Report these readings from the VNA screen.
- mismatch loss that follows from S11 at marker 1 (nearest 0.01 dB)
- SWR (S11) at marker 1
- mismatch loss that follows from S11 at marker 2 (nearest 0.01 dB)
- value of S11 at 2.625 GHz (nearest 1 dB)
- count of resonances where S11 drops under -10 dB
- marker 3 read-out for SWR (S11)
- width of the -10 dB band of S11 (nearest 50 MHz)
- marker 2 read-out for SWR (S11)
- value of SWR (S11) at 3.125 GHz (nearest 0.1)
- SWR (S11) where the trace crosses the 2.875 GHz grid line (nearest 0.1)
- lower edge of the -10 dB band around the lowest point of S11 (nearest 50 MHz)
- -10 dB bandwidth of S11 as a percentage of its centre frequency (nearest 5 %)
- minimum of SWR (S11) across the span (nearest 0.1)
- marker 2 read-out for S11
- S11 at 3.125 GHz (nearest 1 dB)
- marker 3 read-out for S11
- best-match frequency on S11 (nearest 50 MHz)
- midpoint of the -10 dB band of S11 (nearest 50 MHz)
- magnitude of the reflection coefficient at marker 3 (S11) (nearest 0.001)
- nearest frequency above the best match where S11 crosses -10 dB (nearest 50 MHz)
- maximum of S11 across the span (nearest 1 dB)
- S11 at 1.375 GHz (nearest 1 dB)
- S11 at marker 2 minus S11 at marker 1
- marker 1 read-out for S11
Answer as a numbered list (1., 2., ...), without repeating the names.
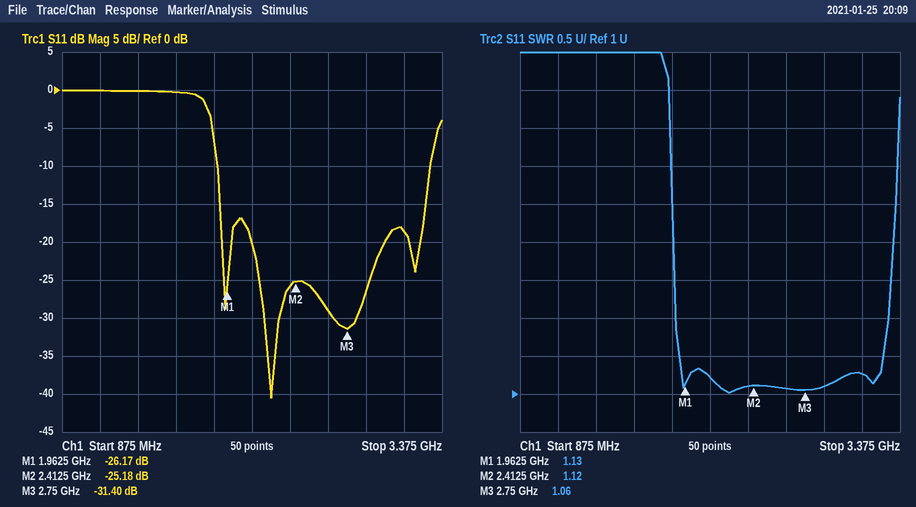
1. 0.01 dB
2. 1.13
3. 0.01 dB
4. -29 dB
5. 4
6. 1.06
7. 1.40 GHz
8. 1.12
9. 1.3
10. 1.1
11. 1.90 GHz
12. 55 %
13. 1.0
14. -25.18 dB
15. -19 dB
16. -31.40 dB
17. 2.25 GHz
18. 2.60 GHz
19. 0.027
20. 3.30 GHz
21. 0 dB
22. 0 dB
23. 0.99 dB
24. -26.17 dB
